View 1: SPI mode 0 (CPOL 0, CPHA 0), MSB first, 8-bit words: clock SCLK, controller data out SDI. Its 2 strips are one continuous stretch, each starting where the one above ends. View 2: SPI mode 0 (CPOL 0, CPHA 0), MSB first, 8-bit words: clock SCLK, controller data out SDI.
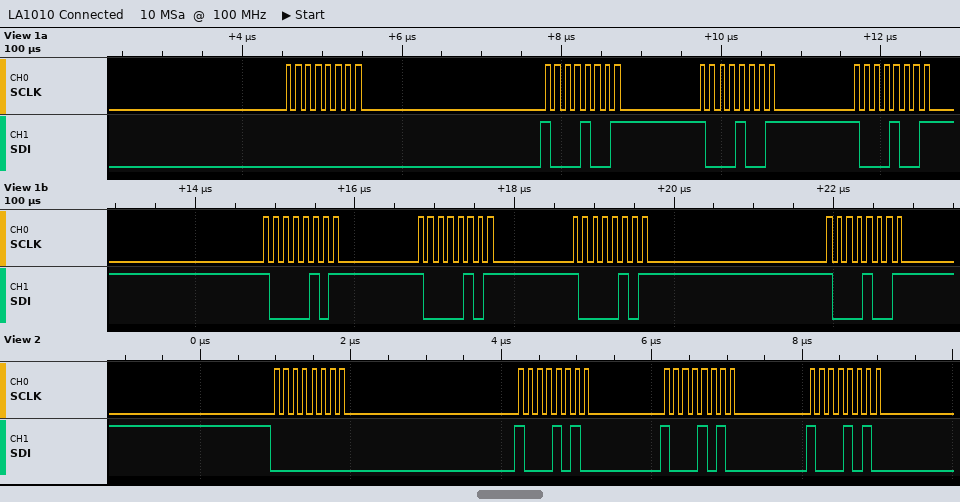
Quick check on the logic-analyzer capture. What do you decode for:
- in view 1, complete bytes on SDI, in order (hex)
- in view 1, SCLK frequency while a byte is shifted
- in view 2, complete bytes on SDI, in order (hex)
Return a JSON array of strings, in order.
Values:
["00 89 89 89 85 85 85 89", "8 MHz", "00 8A 8A 8A"]
